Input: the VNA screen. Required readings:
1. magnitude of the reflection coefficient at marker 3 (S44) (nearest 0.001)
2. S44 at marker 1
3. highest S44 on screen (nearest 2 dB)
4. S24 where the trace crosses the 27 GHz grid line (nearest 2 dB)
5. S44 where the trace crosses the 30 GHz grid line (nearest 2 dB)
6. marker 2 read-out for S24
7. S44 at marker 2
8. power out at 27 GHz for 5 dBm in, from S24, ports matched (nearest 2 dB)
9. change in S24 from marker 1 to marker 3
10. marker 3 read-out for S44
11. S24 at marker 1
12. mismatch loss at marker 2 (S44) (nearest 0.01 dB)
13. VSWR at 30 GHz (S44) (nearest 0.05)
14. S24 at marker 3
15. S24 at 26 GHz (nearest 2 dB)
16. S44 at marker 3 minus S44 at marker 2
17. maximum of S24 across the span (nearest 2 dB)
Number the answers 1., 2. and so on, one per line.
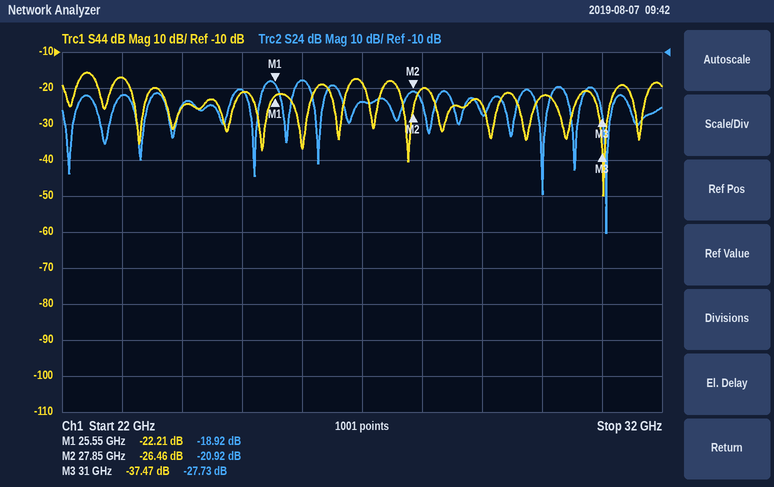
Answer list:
1. 0.013
2. -22.21 dB
3. -16 dB
4. -24 dB
5. -22 dB
6. -20.92 dB
7. -26.46 dB
8. -18 dBm
9. -8.81 dB
10. -37.47 dB
11. -18.92 dB
12. 0.01 dB
13. 1.15
14. -27.73 dB
15. -18 dB
16. -11.01 dB
17. -18 dB
